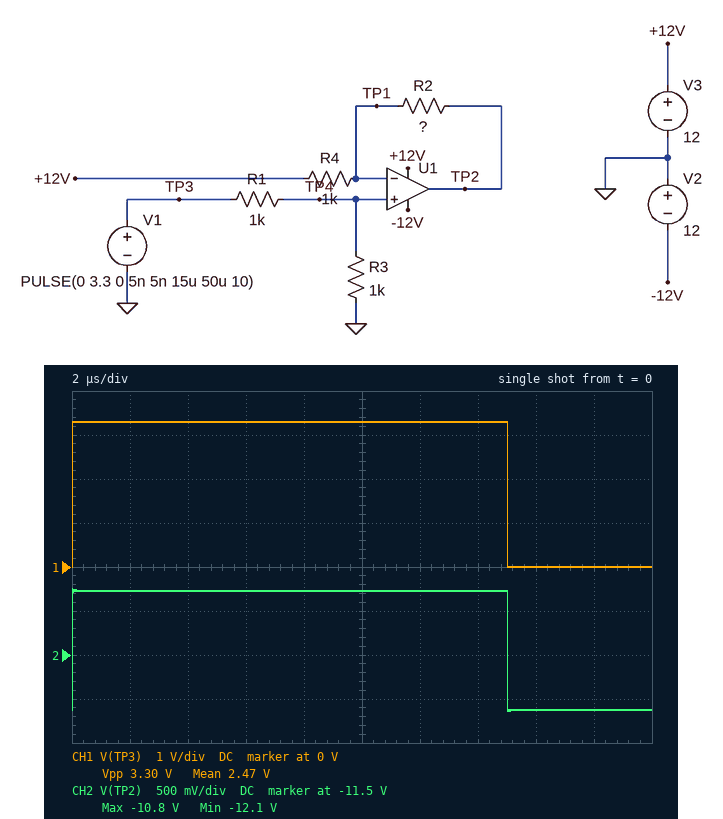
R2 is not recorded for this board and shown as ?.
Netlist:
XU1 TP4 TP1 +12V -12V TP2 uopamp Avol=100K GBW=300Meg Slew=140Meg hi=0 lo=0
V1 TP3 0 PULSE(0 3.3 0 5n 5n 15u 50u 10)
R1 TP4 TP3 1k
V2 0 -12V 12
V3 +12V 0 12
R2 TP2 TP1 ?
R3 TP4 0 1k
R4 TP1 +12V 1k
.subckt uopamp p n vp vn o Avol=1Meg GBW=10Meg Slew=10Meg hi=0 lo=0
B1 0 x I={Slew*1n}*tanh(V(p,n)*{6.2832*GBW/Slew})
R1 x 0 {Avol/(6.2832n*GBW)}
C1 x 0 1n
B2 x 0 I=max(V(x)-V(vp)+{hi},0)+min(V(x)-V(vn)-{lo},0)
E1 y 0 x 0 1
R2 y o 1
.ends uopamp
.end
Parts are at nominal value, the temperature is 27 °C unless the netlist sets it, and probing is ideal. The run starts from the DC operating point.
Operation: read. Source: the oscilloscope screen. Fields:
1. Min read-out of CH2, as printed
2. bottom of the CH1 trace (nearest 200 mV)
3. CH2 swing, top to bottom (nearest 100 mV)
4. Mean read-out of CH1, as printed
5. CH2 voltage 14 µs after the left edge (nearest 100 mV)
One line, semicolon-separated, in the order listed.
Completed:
-12.1 V; 0 V; 1.4 V; 2.47 V; -10.8 V
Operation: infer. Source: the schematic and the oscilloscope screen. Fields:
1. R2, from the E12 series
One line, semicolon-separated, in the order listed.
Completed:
1.2 kΩ
